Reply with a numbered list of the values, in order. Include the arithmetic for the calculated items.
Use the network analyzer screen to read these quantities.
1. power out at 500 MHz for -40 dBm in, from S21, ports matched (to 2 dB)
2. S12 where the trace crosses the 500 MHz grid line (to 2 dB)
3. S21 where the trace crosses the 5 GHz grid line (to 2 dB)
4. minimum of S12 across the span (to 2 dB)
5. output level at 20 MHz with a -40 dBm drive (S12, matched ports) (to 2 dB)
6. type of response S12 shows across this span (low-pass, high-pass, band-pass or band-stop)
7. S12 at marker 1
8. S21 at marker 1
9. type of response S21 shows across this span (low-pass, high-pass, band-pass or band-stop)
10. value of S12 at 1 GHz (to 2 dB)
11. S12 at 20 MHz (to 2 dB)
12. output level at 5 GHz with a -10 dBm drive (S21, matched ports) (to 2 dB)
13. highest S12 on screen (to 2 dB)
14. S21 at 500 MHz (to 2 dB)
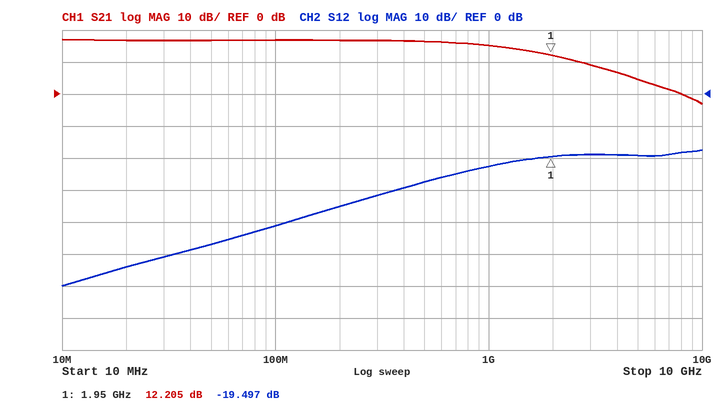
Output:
1. -40 dBm + (16 dB) = -24 dBm
2. -28 dB
3. 4 dB
4. -60 dB
5. -40 dBm + (-54 dB) = -94 dBm
6. high-pass
7. -19.497 dB
8. 12.205 dB
9. low-pass
10. -22 dB
11. -54 dB
12. -10 dBm + (4 dB) = -6 dBm
13. -18 dB
14. 16 dB
